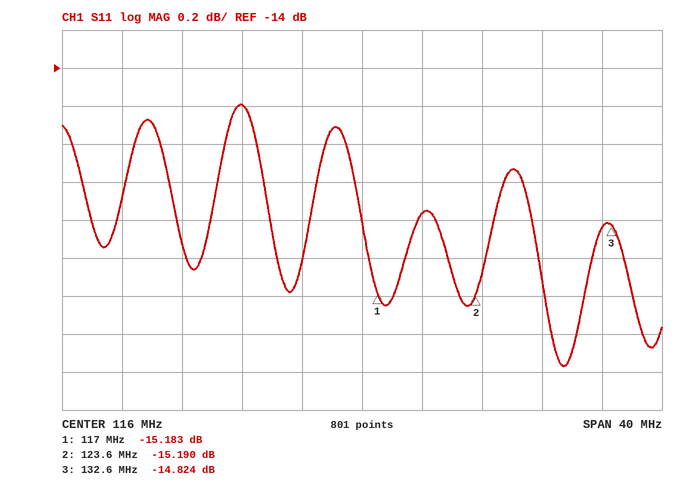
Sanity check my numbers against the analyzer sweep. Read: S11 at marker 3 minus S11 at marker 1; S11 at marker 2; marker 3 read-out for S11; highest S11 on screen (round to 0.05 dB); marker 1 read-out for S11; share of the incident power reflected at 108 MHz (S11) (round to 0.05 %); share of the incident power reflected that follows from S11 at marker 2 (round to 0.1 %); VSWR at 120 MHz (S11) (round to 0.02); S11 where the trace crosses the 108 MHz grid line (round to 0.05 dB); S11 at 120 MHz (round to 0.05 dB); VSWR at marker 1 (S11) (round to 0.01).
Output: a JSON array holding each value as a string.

["0.359 dB", "-15.190 dB", "-14.824 dB", "-14.20 dB", "-15.183 dB", "3.80 %", "3.0 %", "1.44", "-14.20 dB", "-14.75 dB", "1.42"]
